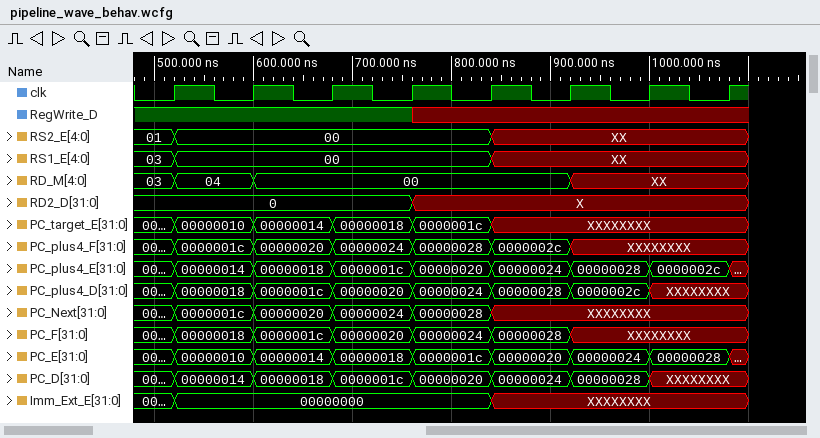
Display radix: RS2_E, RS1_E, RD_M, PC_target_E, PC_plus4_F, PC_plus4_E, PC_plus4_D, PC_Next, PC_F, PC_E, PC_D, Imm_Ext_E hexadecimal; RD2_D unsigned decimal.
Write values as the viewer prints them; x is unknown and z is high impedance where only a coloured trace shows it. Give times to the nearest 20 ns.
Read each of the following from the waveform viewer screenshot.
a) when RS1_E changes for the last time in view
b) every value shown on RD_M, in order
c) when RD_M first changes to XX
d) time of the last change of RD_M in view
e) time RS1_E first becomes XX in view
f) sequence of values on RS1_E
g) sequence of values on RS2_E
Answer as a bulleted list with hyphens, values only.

- 840 ns
- 03, 04, 00, XX
- 920 ns
- 920 ns
- 840 ns
- 03, 00, XX
- 01, 00, XX
